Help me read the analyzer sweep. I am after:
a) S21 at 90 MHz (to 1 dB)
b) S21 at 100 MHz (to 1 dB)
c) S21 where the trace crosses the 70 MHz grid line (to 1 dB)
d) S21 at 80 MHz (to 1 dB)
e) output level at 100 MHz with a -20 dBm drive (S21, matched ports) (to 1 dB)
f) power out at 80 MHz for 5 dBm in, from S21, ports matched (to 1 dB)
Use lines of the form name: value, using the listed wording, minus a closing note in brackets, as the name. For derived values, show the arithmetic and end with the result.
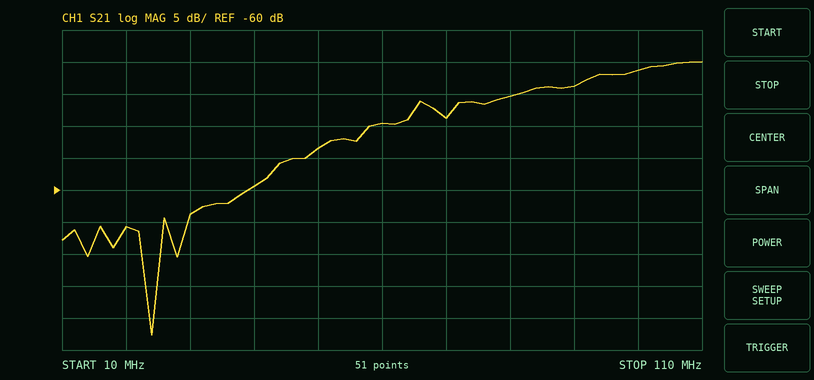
S21 at 90 MHz: -44 dB
S21 at 100 MHz: -41 dB
S21 where the trace crosses the 70 MHz grid line: -49 dB
S21 at 80 MHz: -45 dB
output level at 100 MHz with a -20 dBm drive (S21, matched ports): -20 dBm + (-41 dB) = -61 dBm
power out at 80 MHz for 5 dBm in, from S21, ports matched: 5 dBm + (-45 dB) = -40 dBm
